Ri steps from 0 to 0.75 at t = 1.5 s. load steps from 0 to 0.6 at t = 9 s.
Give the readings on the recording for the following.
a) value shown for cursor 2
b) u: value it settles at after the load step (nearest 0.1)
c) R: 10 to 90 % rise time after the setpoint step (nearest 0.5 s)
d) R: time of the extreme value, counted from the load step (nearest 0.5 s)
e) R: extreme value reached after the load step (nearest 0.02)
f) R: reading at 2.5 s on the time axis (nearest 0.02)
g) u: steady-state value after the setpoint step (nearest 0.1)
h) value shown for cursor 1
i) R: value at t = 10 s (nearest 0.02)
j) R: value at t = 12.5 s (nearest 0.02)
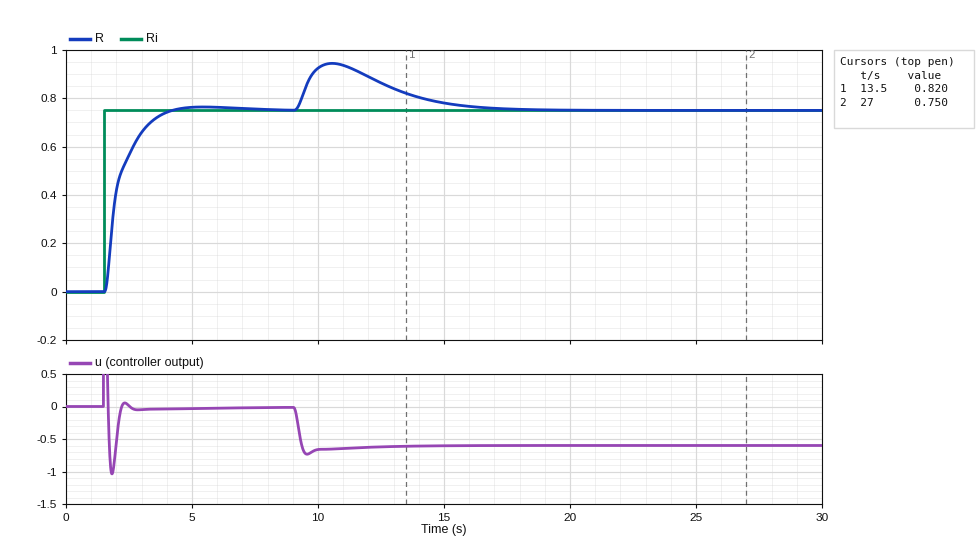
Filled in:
0.750
-0.6
1.5 s
1.5 s
0.94
0.56
0.0
0.820
0.92
0.86
